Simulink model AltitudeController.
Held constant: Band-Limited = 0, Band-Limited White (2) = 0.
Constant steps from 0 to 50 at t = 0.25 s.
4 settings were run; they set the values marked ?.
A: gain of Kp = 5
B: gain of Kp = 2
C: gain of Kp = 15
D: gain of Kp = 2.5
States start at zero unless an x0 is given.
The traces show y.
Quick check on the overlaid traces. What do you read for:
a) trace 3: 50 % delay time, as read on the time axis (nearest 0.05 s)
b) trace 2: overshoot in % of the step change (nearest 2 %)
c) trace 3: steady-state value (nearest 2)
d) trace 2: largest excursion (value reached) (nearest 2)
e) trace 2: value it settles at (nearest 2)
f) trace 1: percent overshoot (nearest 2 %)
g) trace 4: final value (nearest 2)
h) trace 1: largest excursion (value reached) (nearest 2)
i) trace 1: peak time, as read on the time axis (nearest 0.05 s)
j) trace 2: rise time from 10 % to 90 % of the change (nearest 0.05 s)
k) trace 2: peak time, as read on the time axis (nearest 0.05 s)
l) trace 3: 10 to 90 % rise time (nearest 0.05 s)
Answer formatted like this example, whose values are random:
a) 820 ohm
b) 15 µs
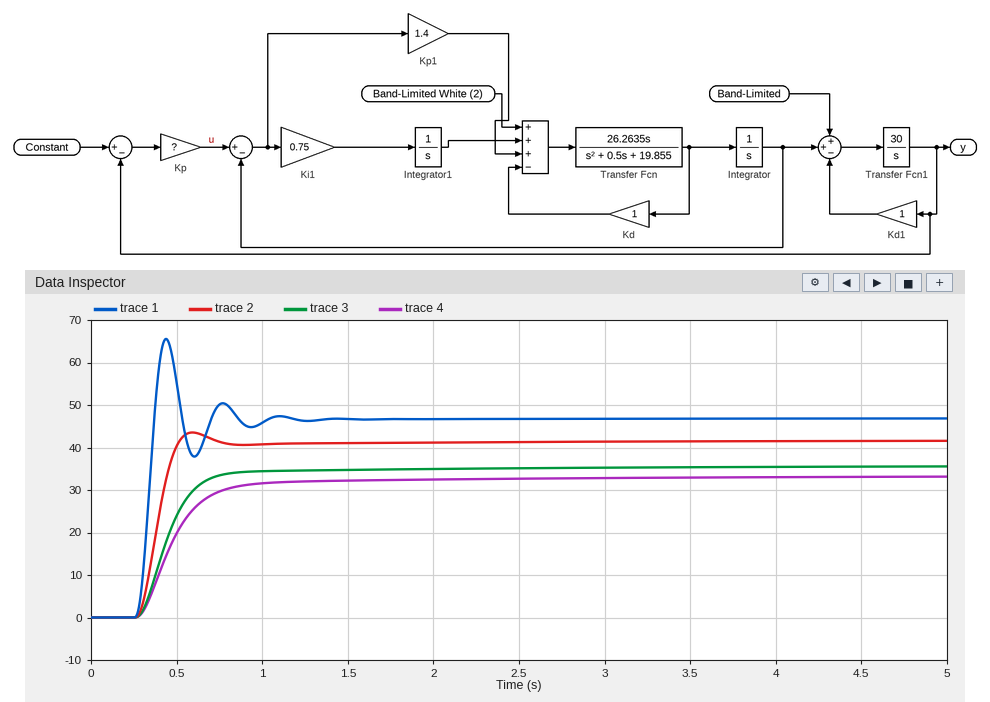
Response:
a) 0.45 s
b) 4 %
c) 36
d) 44
e) 42
f) 40 %
g) 34
h) 66
i) 0.45 s
j) 0.15 s
k) 0.60 s
l) 0.35 s
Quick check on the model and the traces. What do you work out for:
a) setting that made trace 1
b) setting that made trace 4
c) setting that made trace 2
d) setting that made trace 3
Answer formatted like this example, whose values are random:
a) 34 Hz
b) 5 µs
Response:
a) C
b) B
c) A
d) D
